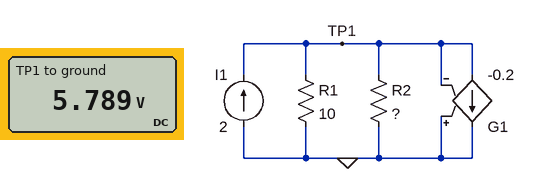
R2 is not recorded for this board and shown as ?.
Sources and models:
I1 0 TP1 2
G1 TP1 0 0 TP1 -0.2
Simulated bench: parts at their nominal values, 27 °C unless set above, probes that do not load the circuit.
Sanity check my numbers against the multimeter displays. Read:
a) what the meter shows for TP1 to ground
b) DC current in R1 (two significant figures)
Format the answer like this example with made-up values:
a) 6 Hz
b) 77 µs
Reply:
a) 5.789 V
b) 580 mA
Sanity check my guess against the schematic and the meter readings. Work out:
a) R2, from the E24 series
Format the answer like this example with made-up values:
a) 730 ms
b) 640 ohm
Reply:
a) 22 Ω
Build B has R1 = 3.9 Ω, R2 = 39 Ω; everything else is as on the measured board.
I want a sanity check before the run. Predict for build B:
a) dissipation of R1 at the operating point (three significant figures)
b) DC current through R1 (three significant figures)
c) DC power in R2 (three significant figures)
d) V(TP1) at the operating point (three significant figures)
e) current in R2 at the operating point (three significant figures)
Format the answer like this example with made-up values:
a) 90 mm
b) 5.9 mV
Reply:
a) 4.41 W
b) 1.06 A
c) 441 mW
d) 4.15 V
e) 106 mA
